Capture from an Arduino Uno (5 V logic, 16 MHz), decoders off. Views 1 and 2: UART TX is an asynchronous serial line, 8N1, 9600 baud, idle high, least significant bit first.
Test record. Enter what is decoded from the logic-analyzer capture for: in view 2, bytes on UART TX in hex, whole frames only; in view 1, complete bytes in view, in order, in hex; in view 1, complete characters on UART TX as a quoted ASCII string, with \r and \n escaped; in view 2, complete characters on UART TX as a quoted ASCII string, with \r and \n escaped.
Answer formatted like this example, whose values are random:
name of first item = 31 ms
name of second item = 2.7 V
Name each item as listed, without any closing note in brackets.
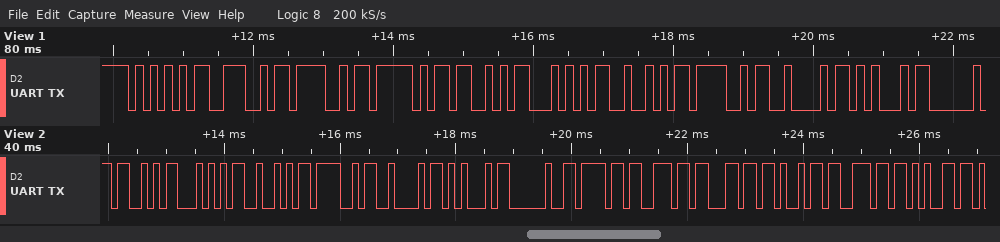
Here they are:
in view 2, bytes on UART TX in hex, whole frames only = 0x53 0x54 0x52 0x4F 0x42 0x45 0x20 0x6F 0x6E 0x6C 0x69 0x6E 0x65
in view 1, complete bytes in view, in order, in hex = 55 4E 4F 5F 53 54 52 4F 42 45
in view 1, complete characters on UART TX as a quoted ASCII string, with \r and \n escaped = "UNO_STROBE"
in view 2, complete characters on UART TX as a quoted ASCII string, with \r and \n escaped = "STROBE online"
